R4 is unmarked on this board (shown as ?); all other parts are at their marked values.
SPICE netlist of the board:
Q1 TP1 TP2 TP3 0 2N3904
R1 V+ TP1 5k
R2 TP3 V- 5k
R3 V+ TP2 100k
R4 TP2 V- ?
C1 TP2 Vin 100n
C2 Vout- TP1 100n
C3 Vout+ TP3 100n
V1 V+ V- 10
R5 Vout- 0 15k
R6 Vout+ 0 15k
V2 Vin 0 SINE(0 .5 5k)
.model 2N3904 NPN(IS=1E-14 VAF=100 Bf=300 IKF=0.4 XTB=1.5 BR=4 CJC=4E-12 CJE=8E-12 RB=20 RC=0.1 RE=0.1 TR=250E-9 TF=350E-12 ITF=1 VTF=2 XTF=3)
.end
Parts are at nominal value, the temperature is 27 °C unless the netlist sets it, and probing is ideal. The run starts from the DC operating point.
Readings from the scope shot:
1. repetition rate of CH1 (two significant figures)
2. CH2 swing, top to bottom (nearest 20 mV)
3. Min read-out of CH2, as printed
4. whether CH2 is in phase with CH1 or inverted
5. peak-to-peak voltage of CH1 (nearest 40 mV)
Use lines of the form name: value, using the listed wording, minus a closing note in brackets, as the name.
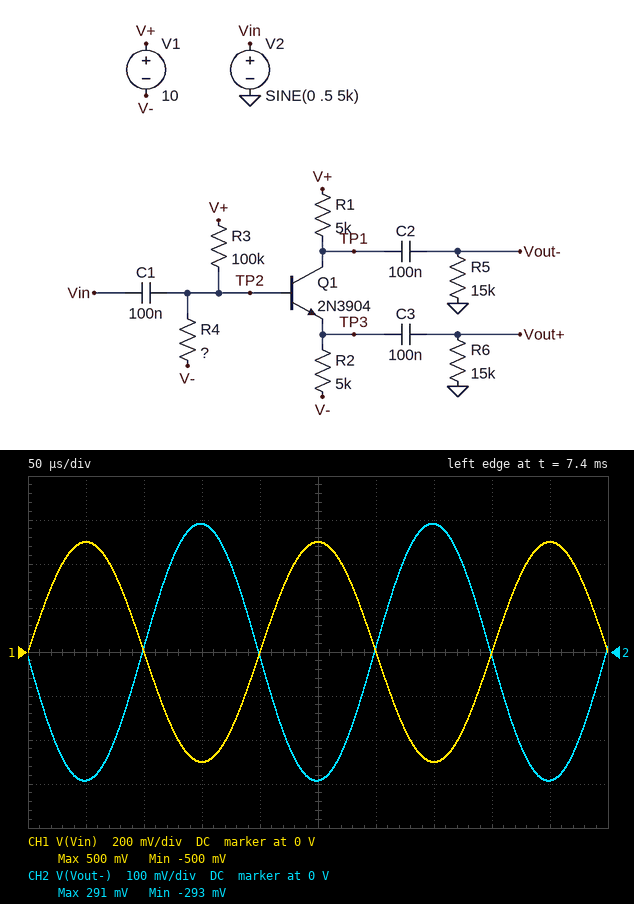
repetition rate of CH1: 5.0 kHz
CH2 swing, top to bottom: 580 mV
Min read-out of CH2, as printed: -293 mV
whether CH2 is in phase with CH1 or inverted: inverted
peak-to-peak voltage of CH1: 1.00 V
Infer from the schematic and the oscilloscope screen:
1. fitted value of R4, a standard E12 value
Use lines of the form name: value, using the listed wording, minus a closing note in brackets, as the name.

fitted value of R4, a standard E12 value: 39 kΩ
